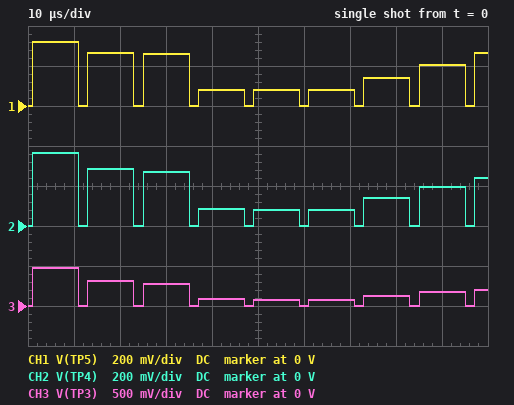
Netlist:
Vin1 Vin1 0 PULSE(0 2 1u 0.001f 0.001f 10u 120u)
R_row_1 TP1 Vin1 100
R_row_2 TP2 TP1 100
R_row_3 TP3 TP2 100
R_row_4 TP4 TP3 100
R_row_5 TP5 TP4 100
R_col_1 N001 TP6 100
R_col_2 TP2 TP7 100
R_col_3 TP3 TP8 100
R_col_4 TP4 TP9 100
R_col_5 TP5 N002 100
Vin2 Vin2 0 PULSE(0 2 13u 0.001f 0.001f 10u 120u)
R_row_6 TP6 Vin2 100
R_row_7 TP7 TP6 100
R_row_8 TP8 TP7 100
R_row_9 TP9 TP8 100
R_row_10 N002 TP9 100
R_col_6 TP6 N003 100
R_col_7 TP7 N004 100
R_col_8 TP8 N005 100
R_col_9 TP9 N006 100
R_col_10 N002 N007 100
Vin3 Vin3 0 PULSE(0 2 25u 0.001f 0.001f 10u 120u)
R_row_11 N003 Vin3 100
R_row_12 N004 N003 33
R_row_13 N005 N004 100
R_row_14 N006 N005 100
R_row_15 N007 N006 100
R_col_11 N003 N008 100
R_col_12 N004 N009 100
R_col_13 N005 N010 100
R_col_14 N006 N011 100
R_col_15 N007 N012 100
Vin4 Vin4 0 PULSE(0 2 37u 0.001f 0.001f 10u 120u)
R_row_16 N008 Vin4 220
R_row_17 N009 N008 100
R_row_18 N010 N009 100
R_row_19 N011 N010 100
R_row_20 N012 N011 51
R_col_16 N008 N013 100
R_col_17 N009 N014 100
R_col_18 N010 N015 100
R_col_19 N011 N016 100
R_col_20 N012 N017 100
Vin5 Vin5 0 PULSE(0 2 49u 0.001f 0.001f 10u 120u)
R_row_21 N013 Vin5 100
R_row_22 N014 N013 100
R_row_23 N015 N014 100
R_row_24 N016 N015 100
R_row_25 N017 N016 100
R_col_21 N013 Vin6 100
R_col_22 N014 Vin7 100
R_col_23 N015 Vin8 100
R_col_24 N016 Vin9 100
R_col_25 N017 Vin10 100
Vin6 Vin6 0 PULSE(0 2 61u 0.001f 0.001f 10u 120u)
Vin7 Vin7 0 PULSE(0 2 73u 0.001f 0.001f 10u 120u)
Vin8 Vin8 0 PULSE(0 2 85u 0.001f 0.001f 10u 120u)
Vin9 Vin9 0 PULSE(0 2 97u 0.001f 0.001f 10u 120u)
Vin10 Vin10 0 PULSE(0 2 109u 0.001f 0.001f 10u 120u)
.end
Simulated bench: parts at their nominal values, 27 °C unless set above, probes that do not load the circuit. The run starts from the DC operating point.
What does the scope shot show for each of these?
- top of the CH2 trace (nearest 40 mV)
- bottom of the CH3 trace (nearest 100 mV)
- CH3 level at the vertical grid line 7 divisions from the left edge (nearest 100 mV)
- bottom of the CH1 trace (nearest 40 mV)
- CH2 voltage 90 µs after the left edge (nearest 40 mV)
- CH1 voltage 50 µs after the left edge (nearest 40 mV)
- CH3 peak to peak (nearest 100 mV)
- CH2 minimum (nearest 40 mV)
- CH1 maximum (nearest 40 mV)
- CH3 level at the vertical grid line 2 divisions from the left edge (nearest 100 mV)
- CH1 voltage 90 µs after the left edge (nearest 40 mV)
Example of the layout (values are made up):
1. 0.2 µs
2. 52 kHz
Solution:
1. 360 mV
2. 0 V
3. 100 mV
4. 0 V
5. 200 mV
6. 80 mV
7. 500 mV
8. 0 V
9. 320 mV
10. 300 mV
11. 200 mV
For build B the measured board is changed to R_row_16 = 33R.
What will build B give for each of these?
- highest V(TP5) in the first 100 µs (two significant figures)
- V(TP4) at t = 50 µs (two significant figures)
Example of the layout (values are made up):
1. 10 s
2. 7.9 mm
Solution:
1. 310 mV
2. 51 mV
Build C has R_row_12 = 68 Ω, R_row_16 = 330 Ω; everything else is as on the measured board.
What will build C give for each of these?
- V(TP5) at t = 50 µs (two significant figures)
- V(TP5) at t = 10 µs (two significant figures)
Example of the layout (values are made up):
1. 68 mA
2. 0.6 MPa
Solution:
1. 85 mV
2. 330 mV
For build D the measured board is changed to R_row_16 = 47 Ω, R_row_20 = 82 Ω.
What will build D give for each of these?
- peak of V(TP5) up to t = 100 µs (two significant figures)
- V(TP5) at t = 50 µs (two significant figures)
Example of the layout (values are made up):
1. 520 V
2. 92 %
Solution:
1. 310 mV
2. 57 mV
